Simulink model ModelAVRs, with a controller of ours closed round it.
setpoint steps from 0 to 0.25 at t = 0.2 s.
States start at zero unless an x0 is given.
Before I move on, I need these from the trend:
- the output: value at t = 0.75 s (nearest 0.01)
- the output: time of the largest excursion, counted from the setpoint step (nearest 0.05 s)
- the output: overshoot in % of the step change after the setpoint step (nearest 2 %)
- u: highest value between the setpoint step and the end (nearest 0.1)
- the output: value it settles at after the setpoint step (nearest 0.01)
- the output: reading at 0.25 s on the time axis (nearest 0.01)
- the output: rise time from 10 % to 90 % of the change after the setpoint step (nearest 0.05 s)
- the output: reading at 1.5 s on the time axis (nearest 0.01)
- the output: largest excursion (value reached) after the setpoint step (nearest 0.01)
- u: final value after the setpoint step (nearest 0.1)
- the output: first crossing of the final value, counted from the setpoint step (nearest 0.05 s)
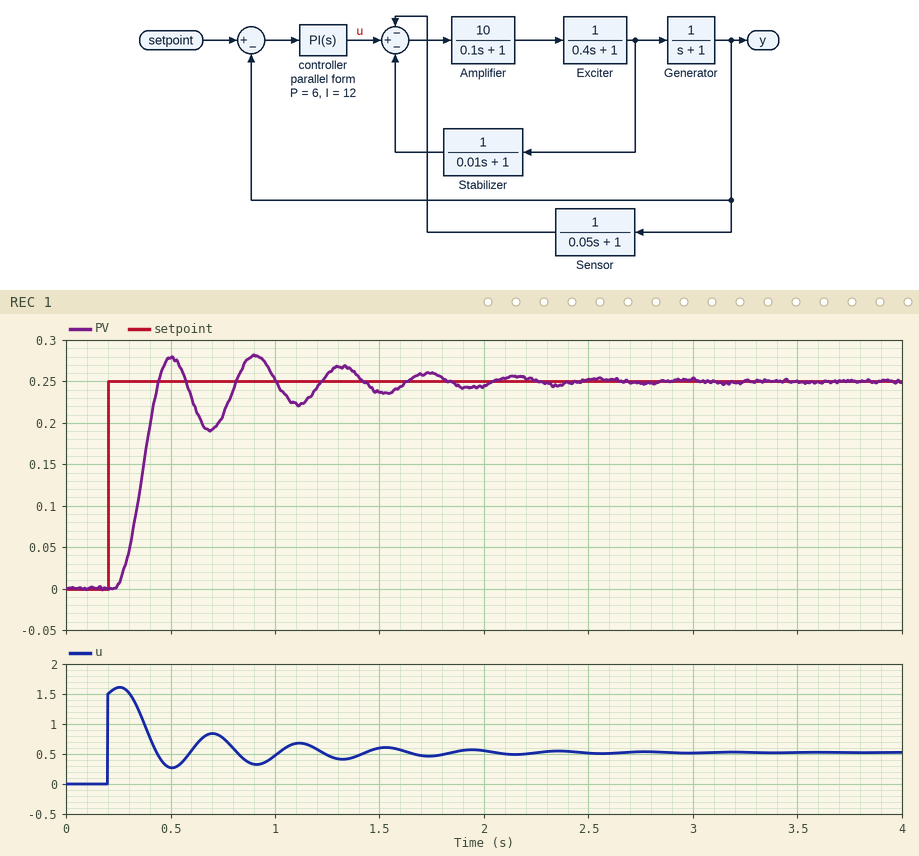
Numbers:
0.21
0.70 s
12 %
1.6
0.25
0.01
0.15 s
0.24
0.28
0.5
0.25 s
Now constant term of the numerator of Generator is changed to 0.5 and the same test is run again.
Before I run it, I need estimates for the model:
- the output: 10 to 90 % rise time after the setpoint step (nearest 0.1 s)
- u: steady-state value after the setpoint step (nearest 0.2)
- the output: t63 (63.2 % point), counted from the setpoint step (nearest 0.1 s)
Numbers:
0.5 s
0.8
0.3 s
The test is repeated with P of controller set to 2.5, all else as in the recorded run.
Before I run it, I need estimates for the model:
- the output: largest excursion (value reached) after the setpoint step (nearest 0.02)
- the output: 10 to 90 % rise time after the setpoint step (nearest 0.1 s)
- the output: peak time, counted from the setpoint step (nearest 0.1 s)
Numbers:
0.28
0.3 s
0.8 s
